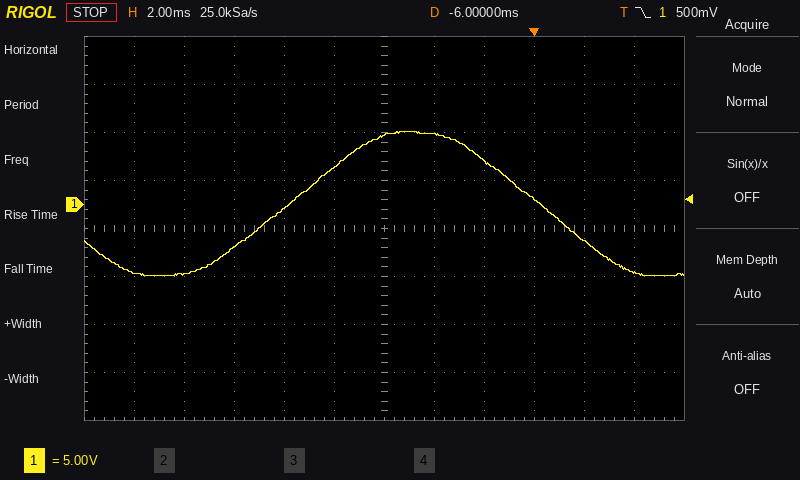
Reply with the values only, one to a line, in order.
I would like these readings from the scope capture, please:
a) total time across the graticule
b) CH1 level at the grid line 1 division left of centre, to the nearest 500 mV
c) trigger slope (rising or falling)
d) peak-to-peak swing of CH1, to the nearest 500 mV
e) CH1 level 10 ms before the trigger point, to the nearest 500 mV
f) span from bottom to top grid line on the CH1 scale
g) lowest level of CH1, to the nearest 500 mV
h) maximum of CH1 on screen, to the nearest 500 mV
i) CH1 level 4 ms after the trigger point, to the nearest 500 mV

24 ms
4.0 V
falling
15.0 V
-500 mV
40 V
-7.5 V
7.5 V
-7.0 V
